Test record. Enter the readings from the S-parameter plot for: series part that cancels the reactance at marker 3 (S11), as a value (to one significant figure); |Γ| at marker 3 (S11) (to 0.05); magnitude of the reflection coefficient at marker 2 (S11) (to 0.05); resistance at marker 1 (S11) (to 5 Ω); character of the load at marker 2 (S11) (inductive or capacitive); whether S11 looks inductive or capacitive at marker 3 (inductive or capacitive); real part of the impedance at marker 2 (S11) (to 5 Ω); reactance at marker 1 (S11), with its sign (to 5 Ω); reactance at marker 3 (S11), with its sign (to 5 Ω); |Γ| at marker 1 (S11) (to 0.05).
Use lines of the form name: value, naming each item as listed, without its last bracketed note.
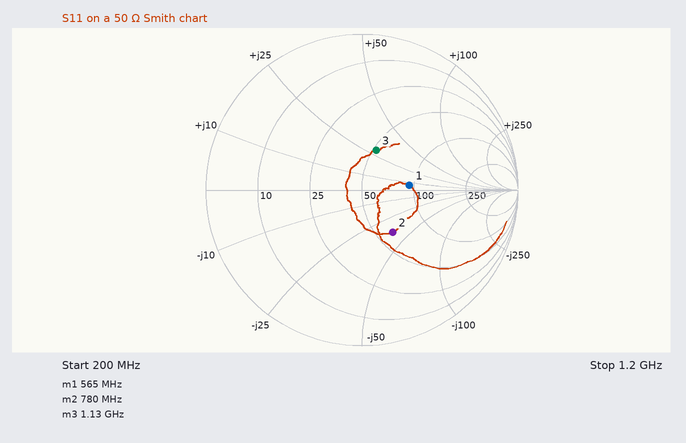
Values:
series part that cancels the reactance at marker 3 (S11), as a value: 5 pF
|Γ| at marker 3 (S11): 0.25
magnitude of the reflection coefficient at marker 2 (S11): 0.35
resistance at marker 1 (S11): 95 Ω
character of the load at marker 2 (S11): capacitive
whether S11 looks inductive or capacitive at marker 3: inductive
real part of the impedance at marker 2 (S11): 60 Ω
reactance at marker 1 (S11), with its sign: +5 Ω
reactance at marker 3 (S11), with its sign: +30 Ω
|Γ| at marker 1 (S11): 0.30
